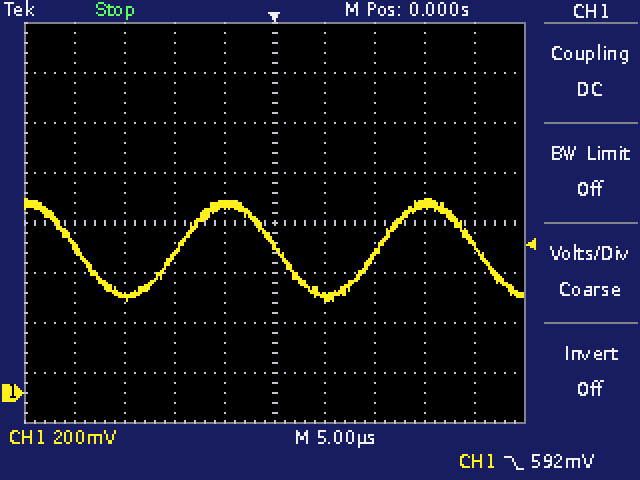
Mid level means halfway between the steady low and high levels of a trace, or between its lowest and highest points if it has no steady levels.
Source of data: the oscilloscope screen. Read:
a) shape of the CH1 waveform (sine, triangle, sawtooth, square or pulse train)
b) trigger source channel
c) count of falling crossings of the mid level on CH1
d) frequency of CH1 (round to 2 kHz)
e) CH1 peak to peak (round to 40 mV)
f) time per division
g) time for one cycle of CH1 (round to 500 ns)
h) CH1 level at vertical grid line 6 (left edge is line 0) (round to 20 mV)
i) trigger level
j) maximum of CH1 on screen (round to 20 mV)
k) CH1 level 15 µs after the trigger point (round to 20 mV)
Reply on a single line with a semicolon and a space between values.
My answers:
sine; CH1; 3; 50 kHz; 400 mV; 5 µs; 20.0 µs; 380 mV; 592 mV; 780 mV; 760 mV
